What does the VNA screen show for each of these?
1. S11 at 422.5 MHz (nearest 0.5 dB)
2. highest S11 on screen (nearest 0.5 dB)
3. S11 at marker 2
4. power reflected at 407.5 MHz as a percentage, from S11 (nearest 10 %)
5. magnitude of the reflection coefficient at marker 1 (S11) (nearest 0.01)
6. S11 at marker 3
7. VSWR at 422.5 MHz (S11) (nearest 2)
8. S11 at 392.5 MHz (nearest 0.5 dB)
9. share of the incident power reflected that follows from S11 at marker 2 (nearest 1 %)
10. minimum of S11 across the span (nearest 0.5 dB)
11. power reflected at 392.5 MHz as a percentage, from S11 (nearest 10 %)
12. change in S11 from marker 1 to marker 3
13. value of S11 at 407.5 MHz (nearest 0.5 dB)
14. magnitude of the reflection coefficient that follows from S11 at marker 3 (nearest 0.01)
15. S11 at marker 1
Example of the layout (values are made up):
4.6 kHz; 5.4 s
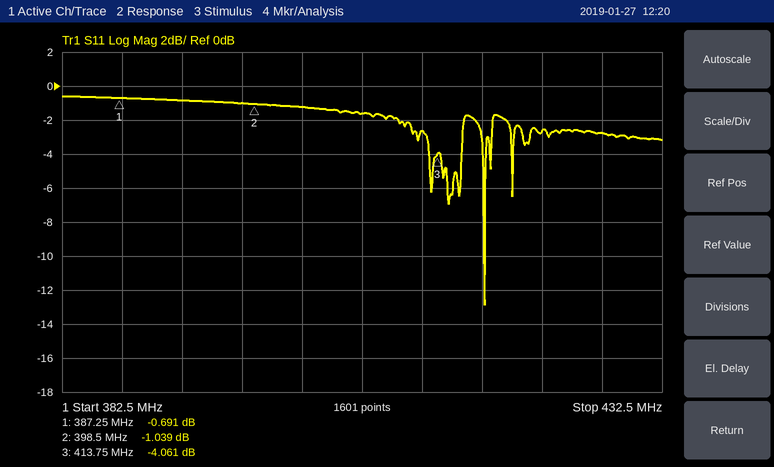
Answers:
-2.5 dB; -0.5 dB; -1.039 dB; 70 %; 0.92; -4.061 dB; 6; -1.0 dB; 79 %; -13.0 dB; 80 %; -3.370 dB; -1.5 dB; 0.63; -0.691 dB
